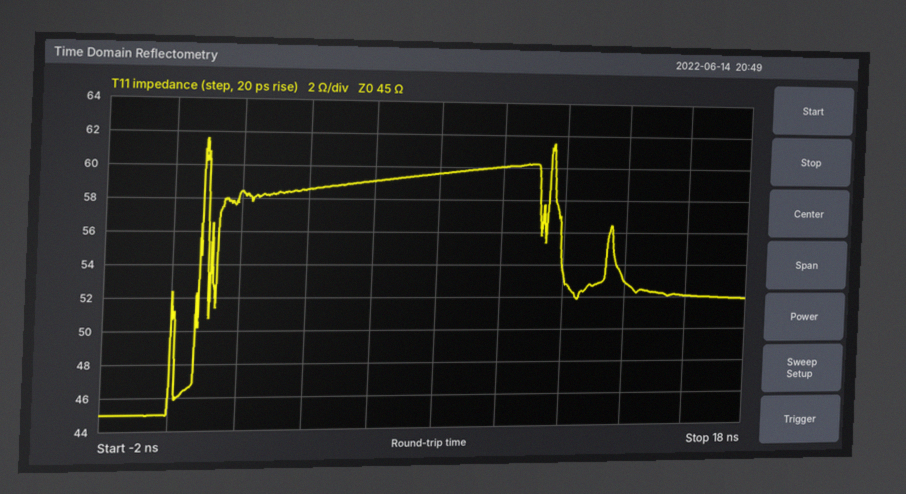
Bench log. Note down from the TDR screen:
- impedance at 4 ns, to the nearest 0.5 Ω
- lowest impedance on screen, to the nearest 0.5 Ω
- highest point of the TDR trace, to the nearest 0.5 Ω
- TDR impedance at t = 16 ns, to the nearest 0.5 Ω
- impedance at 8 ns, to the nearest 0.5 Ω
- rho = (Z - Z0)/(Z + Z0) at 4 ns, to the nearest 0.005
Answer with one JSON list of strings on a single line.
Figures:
["58.5 Ω", "45.0 Ω", "61.5 Ω", "52.0 Ω", "59.5 Ω", "+0.130"]
